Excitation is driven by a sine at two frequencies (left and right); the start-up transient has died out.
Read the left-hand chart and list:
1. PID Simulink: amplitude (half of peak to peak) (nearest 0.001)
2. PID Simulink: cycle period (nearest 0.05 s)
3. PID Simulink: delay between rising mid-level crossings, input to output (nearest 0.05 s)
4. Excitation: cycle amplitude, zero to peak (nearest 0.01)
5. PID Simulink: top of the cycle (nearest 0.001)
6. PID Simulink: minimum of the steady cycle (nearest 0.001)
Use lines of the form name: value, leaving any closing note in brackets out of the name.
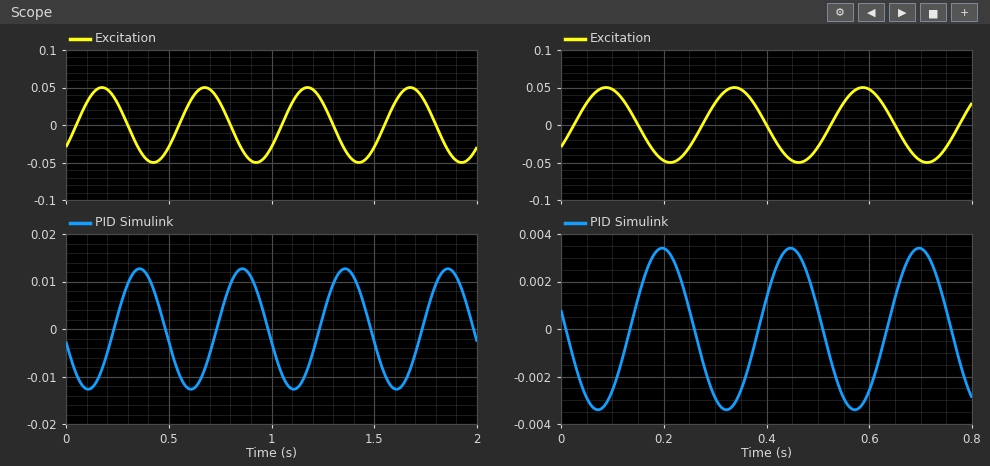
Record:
PID Simulink: amplitude (half of peak to peak): 0.013
PID Simulink: cycle period: 0.50 s
PID Simulink: delay between rising mid-level crossings, input to output: 0.20 s
Excitation: cycle amplitude, zero to peak: 0.05
PID Simulink: top of the cycle: 0.013
PID Simulink: minimum of the steady cycle: -0.013
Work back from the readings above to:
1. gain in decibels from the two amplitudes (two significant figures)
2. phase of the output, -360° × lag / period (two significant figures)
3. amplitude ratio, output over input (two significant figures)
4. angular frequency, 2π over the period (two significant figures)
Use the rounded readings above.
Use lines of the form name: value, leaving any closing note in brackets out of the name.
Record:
gain in decibels from the two amplitudes: -12 dB
phase of the output, -360° × lag / period: -140°
amplitude ratio, output over input: 0.26
angular frequency, 2π over the period: 13 rad/s
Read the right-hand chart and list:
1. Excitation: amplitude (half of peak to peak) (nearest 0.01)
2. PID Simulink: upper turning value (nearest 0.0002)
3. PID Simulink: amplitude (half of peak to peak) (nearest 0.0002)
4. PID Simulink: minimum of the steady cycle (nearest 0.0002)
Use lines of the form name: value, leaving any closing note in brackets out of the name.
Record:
Excitation: amplitude (half of peak to peak): 0.05
PID Simulink: upper turning value: 0.0034
PID Simulink: amplitude (half of peak to peak): 0.0034
PID Simulink: minimum of the steady cycle: -0.0034
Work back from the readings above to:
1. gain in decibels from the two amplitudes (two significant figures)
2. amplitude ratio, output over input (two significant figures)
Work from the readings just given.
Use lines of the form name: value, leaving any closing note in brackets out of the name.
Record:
gain in decibels from the two amplitudes: -23 dB
amplitude ratio, output over input: 0.068
